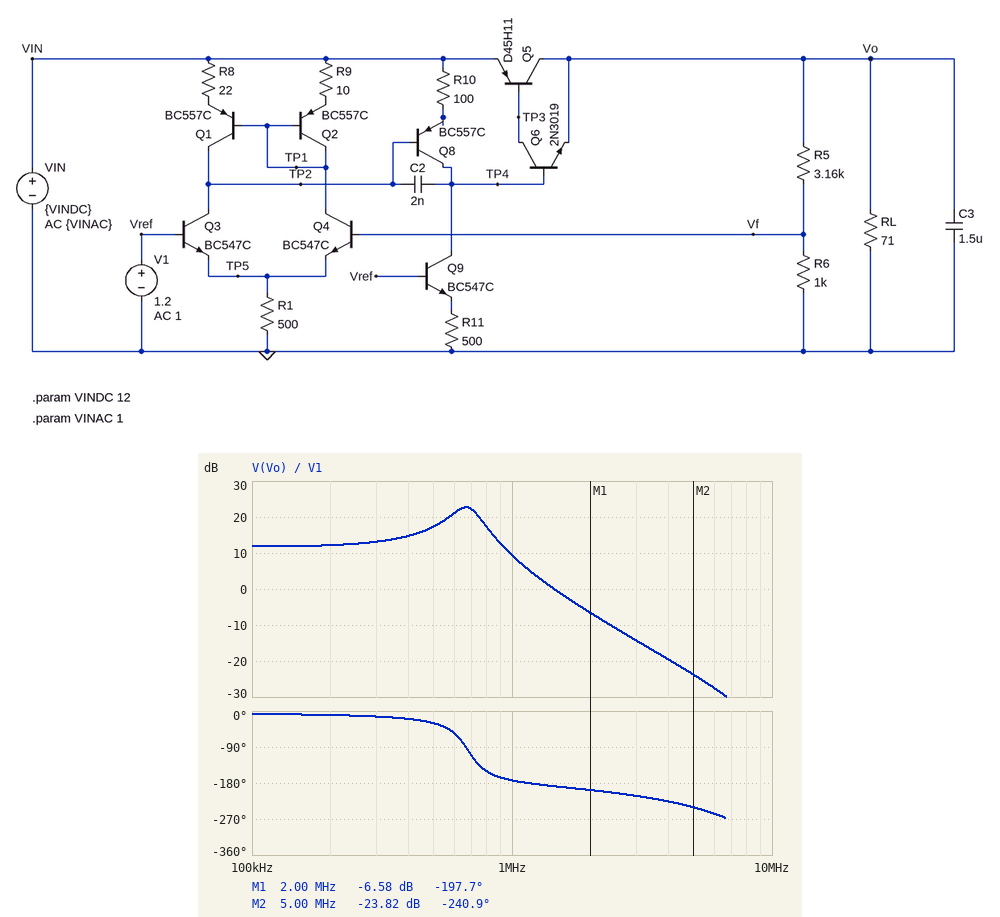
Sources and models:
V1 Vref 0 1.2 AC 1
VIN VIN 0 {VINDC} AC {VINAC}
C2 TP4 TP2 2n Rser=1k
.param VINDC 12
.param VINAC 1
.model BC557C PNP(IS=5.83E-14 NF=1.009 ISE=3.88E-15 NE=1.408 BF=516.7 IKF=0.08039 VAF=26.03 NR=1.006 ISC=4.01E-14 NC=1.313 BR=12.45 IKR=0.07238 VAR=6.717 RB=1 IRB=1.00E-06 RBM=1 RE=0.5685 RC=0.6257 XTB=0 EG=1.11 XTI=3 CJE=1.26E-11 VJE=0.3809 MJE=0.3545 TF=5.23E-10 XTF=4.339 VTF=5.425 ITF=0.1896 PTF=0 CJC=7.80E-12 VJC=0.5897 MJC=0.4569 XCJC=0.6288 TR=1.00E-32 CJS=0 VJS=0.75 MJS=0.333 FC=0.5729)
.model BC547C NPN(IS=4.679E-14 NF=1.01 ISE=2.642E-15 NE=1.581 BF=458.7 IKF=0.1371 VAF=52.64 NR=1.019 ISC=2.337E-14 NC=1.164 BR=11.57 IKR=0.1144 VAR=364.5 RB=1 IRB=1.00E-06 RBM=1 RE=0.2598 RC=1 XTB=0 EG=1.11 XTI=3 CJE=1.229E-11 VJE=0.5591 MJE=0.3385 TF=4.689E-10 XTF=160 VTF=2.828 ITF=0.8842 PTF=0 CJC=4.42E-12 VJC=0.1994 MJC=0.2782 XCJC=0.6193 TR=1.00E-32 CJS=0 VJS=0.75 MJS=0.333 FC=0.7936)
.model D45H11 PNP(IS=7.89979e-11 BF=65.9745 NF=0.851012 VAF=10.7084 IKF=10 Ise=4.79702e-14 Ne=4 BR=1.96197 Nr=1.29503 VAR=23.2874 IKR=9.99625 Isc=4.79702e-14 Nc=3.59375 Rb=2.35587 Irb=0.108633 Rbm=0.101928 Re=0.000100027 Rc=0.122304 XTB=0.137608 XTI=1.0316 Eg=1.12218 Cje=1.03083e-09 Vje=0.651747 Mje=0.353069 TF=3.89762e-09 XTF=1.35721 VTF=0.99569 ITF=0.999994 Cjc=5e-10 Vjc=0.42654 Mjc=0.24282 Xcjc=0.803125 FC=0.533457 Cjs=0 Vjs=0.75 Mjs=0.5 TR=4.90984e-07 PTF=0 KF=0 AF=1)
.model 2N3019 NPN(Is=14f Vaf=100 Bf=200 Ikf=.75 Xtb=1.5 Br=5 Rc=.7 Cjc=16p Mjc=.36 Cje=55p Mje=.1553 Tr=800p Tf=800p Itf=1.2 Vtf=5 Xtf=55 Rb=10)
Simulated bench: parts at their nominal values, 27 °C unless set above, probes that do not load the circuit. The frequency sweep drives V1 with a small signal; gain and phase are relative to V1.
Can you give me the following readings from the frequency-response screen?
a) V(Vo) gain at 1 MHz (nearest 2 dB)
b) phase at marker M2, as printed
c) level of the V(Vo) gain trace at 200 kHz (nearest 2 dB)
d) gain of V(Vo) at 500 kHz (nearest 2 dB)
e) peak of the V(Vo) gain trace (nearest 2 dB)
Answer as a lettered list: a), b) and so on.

a) 10 dB
b) -240.9 deg
c) 12 dB
d) 18 dB
e) 22 dB
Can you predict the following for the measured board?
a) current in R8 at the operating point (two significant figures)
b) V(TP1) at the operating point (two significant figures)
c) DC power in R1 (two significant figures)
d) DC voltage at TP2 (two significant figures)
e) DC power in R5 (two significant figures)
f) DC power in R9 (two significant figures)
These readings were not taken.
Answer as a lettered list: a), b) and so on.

a) 540 µA
b) 11 V
c) 720 µW
d) 11 V
e) 4.6 mW
f) 4.3 µW
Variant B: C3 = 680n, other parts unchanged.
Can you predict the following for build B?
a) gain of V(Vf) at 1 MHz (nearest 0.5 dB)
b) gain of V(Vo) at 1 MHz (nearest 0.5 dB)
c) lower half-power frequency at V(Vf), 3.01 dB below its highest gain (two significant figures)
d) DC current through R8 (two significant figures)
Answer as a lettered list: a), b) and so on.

a) 19.5 dB
b) 32.0 dB
c) 970 kHz
d) 540 µA
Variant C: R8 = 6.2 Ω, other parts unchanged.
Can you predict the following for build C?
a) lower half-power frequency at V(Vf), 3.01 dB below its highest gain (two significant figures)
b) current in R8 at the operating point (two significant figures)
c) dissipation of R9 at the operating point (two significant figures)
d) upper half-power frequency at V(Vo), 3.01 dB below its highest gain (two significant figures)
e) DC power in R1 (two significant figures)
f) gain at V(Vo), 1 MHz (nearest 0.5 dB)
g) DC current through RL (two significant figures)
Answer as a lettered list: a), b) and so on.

a) 650 kHz
b) 620 µA
c) 3.3 µW
d) 810 kHz
e) 710 µW
f) 12.5 dB
g) 70 mA
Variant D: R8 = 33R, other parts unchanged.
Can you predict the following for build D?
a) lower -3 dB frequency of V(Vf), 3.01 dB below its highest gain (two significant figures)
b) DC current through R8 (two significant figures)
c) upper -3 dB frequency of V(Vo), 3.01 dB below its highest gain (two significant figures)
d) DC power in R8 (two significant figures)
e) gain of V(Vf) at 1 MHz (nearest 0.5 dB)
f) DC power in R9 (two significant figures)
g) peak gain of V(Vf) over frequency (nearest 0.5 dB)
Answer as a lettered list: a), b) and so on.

a) 520 kHz
b) 500 µA
c) 730 kHz
d) 8.1 µW
e) -5.0 dB
f) 4.9 µW
g) 9.0 dB
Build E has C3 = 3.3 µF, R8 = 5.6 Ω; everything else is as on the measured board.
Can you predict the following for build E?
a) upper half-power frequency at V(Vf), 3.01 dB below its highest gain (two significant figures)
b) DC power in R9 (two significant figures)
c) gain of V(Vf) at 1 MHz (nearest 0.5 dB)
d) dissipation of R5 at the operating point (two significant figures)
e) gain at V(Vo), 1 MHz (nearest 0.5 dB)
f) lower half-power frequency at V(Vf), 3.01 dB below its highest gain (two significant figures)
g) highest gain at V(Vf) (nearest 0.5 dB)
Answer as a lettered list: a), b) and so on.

a) 560 kHz
b) 3.2 µW
c) -11.0 dB
d) 4.5 mW
e) 1.5 dB
f) 340 kHz
g) 7.0 dB
